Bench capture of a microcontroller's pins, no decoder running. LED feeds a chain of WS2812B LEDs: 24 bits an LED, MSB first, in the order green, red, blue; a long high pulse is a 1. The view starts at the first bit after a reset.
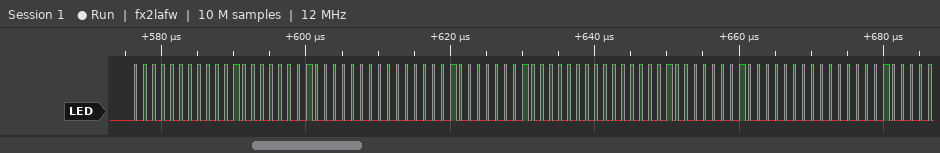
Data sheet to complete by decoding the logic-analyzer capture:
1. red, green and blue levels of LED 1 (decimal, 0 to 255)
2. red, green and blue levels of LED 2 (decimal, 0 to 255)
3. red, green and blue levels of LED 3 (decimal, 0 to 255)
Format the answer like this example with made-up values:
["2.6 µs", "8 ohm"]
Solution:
["16, 0, 16", "16, 0, 16", "16, 0, 16"]
